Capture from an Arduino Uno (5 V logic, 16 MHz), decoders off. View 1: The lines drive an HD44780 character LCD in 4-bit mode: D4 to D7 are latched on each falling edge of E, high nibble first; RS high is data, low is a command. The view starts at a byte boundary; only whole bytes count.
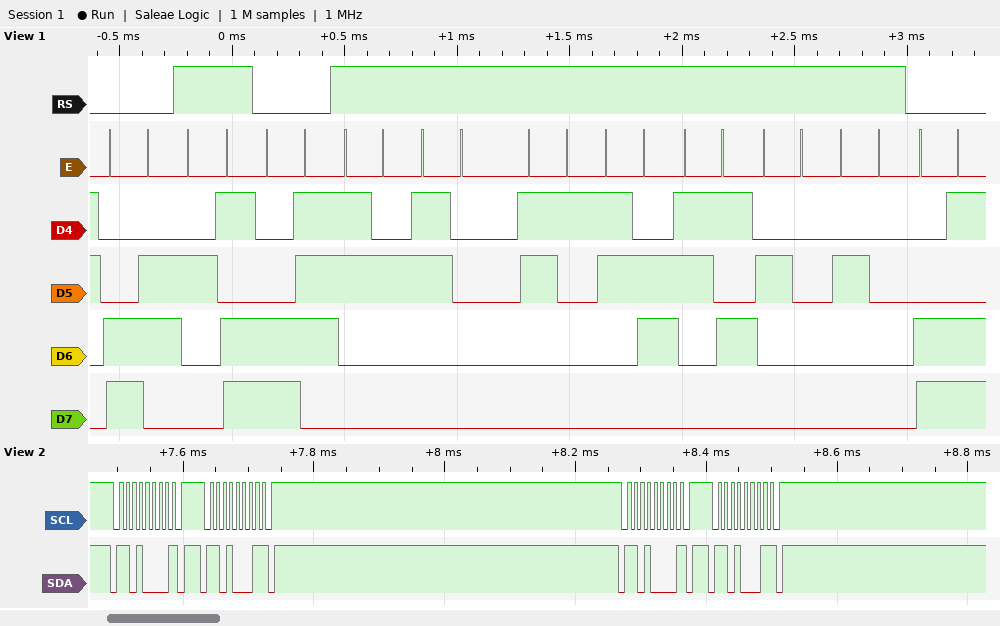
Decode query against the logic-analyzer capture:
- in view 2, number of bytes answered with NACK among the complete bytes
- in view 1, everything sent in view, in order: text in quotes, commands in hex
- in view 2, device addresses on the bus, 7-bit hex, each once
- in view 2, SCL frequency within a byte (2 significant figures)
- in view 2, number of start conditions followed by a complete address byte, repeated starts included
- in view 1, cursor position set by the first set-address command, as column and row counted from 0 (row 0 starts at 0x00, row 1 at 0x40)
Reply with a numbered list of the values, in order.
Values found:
1. 4
2. 0xC6 "-" 0xC7 "20165  " 0xCD
3. 0x68
4. 100 kHz
5. 4
6. column 6, row 1
